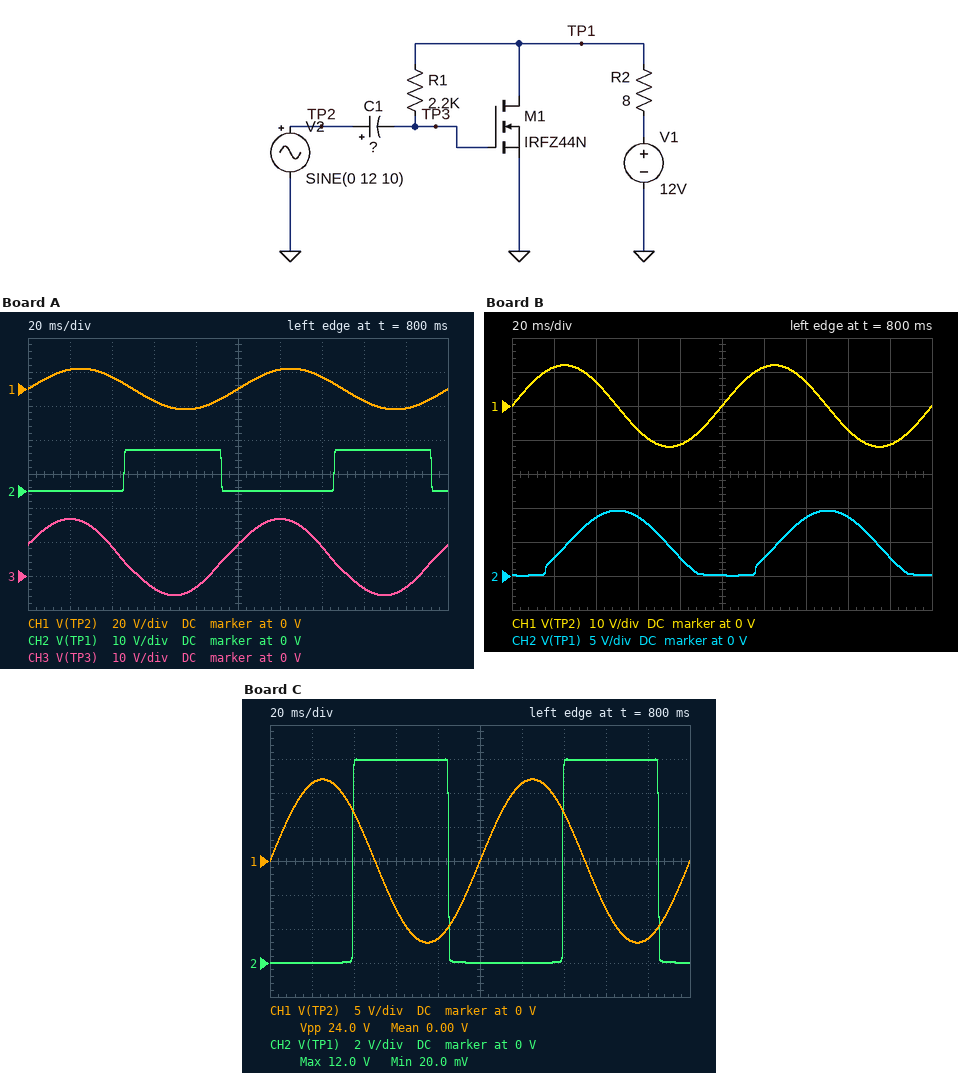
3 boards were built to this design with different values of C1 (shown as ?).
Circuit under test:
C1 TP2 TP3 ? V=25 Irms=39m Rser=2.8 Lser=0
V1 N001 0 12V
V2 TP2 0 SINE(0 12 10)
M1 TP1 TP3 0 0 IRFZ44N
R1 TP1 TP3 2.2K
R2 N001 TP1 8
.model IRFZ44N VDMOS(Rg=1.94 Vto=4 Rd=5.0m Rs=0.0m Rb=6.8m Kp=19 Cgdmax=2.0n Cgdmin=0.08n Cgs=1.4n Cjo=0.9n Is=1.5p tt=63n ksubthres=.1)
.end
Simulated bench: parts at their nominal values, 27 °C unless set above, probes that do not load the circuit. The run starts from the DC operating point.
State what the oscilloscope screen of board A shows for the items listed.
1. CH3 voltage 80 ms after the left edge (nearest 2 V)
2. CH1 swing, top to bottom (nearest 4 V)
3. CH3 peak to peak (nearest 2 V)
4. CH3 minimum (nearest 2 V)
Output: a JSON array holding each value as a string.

["-4 V", "24 V", "22 V", "-6 V"]
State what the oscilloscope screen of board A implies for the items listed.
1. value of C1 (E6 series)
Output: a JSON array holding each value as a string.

["33 µF"]
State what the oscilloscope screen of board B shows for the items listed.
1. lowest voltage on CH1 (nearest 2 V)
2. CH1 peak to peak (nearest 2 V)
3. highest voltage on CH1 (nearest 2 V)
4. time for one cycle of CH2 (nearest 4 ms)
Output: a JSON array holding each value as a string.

["-12 V", "24 V", "12 V", "100 ms"]
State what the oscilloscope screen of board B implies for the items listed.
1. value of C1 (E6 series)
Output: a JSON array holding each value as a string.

["3.3 µF"]
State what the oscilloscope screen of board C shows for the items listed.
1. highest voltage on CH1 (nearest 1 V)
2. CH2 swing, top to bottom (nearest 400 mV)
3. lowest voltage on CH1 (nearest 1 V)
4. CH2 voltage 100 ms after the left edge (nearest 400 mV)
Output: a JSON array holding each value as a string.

["12 V", "12.0 V", "-12 V", "0 V"]
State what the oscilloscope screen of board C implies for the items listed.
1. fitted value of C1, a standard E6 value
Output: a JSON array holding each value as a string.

["15 µF"]
